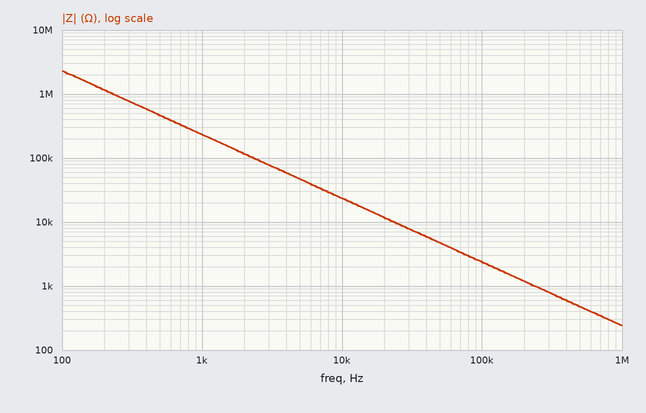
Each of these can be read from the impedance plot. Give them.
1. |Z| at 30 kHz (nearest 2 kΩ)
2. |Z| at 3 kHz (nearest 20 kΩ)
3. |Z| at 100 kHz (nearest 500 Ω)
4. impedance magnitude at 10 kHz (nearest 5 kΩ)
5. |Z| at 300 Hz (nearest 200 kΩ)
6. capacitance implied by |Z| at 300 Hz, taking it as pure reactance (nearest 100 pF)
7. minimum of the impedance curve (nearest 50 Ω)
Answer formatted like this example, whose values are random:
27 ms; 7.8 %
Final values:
8 kΩ; 80 kΩ; 2.5 kΩ; 25 kΩ; 800 kΩ; 700 pF; 250 Ω
